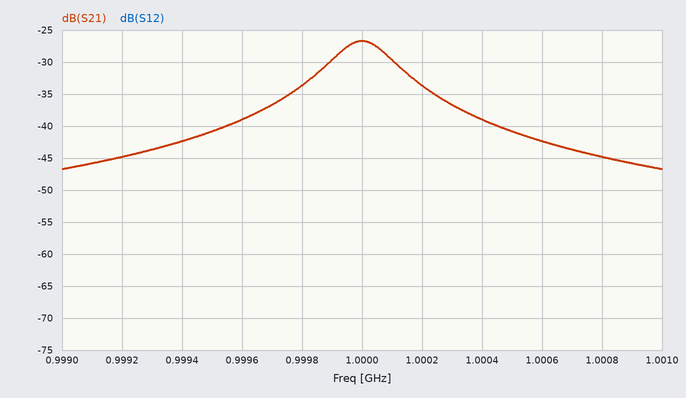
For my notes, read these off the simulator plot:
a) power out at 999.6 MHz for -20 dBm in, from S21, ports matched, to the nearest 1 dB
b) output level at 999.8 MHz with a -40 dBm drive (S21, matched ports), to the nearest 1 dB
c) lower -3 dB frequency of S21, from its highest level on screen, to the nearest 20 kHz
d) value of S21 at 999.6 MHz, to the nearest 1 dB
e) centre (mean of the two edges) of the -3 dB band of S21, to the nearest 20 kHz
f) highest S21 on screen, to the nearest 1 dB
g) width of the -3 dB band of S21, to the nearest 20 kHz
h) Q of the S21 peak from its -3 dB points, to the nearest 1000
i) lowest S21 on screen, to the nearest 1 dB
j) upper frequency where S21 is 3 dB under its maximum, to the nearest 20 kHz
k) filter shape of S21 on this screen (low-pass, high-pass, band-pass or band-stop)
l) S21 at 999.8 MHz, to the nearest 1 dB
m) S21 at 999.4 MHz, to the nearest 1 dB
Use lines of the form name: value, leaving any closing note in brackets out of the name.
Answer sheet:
power out at 999.6 MHz for -20 dBm in, from S21, ports matched, to the nearest 1 dB: -59 dBm
output level at 999.8 MHz with a -40 dBm drive (S21, matched ports), to the nearest 1 dB: -74 dBm
lower -3 dB frequency of S21, from its highest level on screen, to the nearest 20 kHz: 999.90 MHz
value of S21 at 999.6 MHz, to the nearest 1 dB: -39 dB
centre (mean of the two edges) of the -3 dB band of S21, to the nearest 20 kHz: 1.00000 GHz
highest S21 on screen, to the nearest 1 dB: -27 dB
width of the -3 dB band of S21, to the nearest 20 kHz: 200 kHz
Q of the S21 peak from its -3 dB points, to the nearest 1000: 5000
lowest S21 on screen, to the nearest 1 dB: -47 dB
upper frequency where S21 is 3 dB under its maximum, to the nearest 20 kHz: 1.00010 GHz
filter shape of S21 on this screen: band-pass
S21 at 999.8 MHz, to the nearest 1 dB: -34 dB
S21 at 999.4 MHz, to the nearest 1 dB: -42 dB
